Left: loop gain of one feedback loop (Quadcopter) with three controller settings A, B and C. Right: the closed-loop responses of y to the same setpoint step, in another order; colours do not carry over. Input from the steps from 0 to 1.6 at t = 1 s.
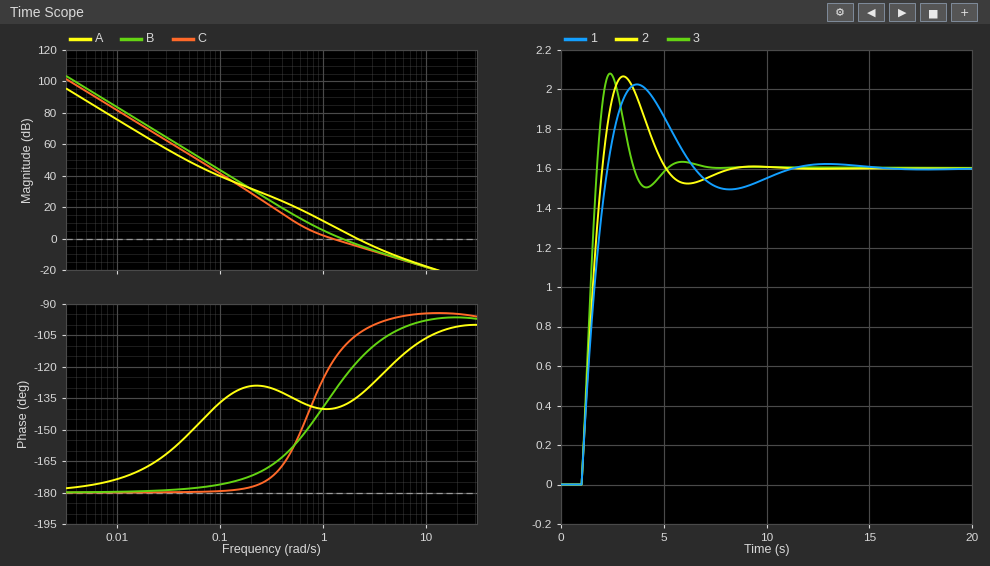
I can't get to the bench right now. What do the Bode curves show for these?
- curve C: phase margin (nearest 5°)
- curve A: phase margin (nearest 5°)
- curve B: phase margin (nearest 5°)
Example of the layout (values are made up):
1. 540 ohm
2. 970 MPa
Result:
1. 60°
2. 45°
3. 55°
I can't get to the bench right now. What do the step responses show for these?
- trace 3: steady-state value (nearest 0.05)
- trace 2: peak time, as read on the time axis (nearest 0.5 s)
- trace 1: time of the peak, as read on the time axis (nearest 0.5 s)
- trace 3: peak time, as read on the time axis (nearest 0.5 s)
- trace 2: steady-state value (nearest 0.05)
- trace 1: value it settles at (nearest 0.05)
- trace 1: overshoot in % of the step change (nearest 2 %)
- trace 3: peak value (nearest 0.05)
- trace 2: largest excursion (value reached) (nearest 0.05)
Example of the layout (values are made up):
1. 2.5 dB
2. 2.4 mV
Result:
1. 1.60
2. 3.0 s
3. 3.5 s
4. 2.5 s
5. 1.60
6. 1.60
7. 26 %
8. 2.10
9. 2.05
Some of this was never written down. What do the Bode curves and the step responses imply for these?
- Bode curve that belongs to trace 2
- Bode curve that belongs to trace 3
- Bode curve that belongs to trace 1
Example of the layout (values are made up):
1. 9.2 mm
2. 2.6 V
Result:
1. B
2. A
3. C
